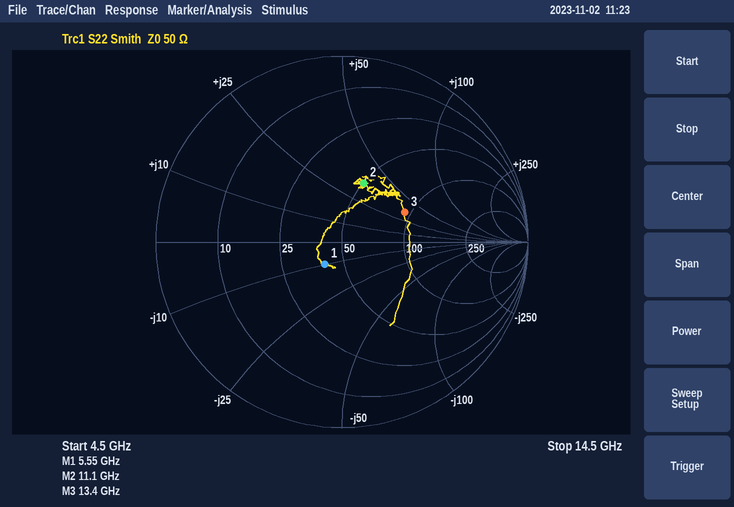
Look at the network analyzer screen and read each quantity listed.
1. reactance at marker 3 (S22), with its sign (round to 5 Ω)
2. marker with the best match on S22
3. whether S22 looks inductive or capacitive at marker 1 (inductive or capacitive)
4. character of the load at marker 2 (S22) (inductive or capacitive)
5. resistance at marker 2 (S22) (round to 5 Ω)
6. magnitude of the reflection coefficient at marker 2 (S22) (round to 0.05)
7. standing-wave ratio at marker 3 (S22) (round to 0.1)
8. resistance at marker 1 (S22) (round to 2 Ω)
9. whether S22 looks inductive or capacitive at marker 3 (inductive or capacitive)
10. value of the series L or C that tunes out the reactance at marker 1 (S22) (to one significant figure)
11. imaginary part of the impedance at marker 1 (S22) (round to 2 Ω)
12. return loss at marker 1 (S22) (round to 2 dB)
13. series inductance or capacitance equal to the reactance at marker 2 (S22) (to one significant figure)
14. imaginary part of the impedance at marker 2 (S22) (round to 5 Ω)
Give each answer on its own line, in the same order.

+35 Ω
marker 1
capacitive
inductive
50 Ω
0.35
2.2
40 Ω
inductive
300 pH
-10 Ω
16 dB
500 pH
+35 Ω
